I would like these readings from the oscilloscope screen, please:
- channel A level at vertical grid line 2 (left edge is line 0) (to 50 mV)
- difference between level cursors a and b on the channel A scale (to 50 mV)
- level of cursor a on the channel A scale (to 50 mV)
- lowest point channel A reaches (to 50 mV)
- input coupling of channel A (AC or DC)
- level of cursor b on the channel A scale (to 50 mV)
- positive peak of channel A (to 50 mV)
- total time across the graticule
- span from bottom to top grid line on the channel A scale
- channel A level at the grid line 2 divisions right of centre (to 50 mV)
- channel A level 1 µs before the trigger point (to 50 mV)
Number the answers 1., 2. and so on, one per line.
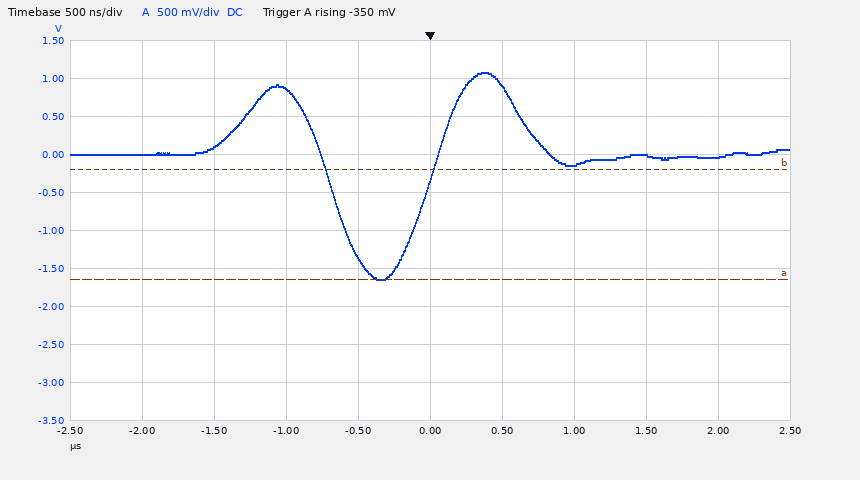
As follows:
1. 100 mV
2. 1.45 V
3. -1.65 V
4. -1.65 V
5. DC
6. -200 mV
7. 1.10 V
8. 5 µs
9. 5 V
10. -150 mV
11. 850 mV
